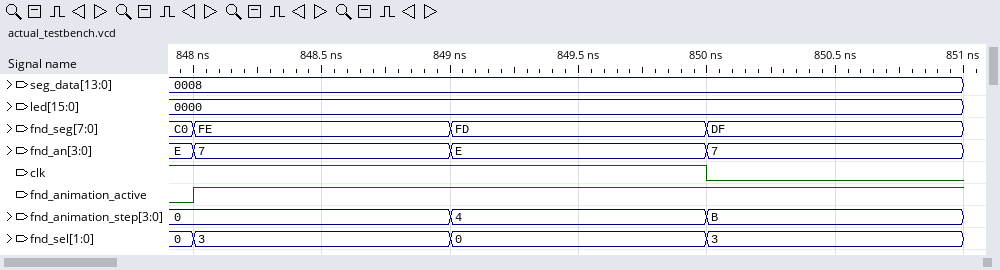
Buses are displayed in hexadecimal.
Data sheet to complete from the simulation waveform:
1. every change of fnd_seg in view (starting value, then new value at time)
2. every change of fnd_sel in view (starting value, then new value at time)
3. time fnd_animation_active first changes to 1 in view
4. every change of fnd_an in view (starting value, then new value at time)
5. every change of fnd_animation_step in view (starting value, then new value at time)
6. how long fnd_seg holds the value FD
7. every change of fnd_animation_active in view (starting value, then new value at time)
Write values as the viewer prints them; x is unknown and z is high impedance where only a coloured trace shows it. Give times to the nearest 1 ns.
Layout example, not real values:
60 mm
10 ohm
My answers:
C0, FE at 848 ns, FD at 849 ns, DF at 850 ns
0, 3 at 848 ns, 0 at 849 ns, 3 at 850 ns
848 ns
E, 7 at 848 ns, E at 849 ns, 7 at 850 ns
0, 4 at 849 ns, B at 850 ns
1 ns
0, 1 at 848 ns
